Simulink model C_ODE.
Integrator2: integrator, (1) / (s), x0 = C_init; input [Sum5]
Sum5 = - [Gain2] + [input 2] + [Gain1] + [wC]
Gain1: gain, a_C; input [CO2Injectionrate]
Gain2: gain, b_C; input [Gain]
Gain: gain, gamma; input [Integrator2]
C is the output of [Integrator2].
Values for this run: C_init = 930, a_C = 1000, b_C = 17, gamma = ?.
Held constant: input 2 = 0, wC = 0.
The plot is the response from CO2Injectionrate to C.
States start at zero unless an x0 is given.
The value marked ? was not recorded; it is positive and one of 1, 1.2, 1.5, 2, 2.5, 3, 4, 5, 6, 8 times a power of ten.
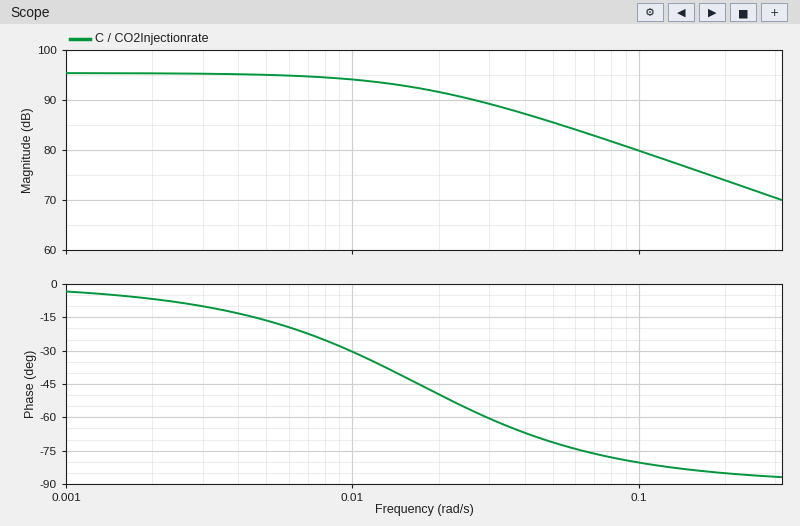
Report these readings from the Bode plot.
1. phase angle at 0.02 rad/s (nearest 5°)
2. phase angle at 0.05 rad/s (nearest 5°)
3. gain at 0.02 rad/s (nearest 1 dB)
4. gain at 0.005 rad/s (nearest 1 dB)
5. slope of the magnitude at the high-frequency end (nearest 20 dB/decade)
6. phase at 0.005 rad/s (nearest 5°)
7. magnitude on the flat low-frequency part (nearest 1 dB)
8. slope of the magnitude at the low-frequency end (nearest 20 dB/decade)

-50°
-70°
92 dB
95 dB
-20 dB/decade
-15°
95 dB
0 dB/decade
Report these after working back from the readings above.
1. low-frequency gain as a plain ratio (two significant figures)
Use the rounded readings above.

56000
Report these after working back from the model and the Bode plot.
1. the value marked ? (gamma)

0.001
